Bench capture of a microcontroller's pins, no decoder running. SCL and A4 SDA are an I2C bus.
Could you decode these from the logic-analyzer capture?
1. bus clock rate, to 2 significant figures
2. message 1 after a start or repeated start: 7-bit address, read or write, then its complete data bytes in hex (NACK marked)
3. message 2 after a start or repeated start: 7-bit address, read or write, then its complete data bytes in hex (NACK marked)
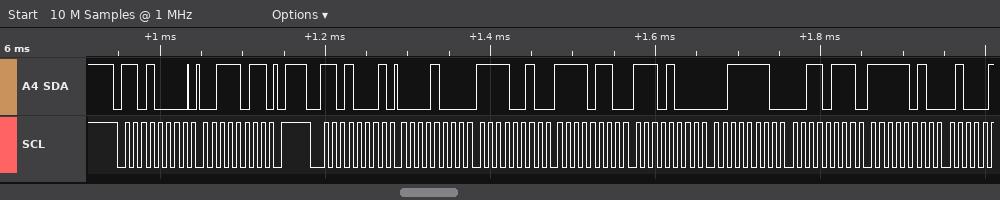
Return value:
100 kHz
0x68 write: 3B
0x68 read: 08 F2 F6 E8 3E 37 FA
